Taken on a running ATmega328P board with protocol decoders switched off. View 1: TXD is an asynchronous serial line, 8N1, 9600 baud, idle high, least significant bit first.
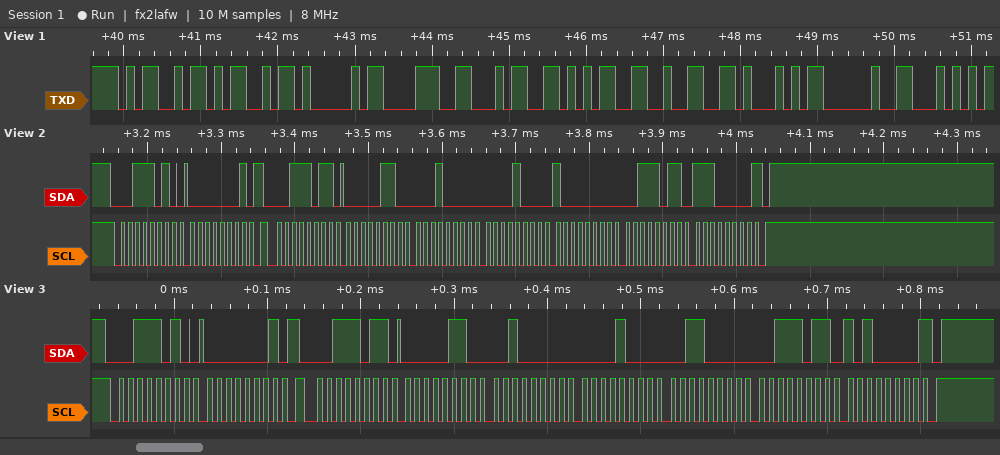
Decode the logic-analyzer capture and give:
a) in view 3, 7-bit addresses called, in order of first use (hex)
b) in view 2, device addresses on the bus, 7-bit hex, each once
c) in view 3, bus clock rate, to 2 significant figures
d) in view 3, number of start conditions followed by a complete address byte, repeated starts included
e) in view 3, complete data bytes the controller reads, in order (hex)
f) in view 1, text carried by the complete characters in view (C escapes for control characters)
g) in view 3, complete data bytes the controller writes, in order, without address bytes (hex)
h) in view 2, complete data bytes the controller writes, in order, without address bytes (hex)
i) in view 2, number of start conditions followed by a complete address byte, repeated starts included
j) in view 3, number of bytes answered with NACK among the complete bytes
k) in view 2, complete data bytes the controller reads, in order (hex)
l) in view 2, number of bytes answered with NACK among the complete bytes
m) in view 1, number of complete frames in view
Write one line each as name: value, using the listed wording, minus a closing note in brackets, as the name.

in view 3, 7-bit addresses called, in order of first use: 0x1D
in view 2, device addresses on the bus, 7-bit hex, each once: 0x1D
in view 3, bus clock rate, to 2 significant figures: 100 kHz
in view 3, number of start conditions followed by a complete address byte, repeated starts included: 2
in view 3, complete data bytes the controller reads, in order: 06 20 08 30 3B A0
in view 1, text carried by the complete characters in view: "MMA8452Q T"
in view 3, complete data bytes the controller writes, in order, without address bytes: 01
in view 2, complete data bytes the controller writes, in order, without address bytes: 01
in view 2, number of start conditions followed by a complete address byte, repeated starts included: 2
in view 3, number of bytes answered with NACK among the complete bytes: 1
in view 2, complete data bytes the controller reads, in order: 06 10 08 80 3B E0
in view 2, number of bytes answered with NACK among the complete bytes: 1
in view 1, number of complete frames in view: 10
